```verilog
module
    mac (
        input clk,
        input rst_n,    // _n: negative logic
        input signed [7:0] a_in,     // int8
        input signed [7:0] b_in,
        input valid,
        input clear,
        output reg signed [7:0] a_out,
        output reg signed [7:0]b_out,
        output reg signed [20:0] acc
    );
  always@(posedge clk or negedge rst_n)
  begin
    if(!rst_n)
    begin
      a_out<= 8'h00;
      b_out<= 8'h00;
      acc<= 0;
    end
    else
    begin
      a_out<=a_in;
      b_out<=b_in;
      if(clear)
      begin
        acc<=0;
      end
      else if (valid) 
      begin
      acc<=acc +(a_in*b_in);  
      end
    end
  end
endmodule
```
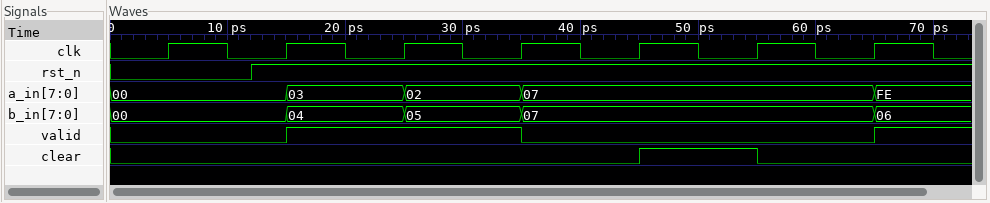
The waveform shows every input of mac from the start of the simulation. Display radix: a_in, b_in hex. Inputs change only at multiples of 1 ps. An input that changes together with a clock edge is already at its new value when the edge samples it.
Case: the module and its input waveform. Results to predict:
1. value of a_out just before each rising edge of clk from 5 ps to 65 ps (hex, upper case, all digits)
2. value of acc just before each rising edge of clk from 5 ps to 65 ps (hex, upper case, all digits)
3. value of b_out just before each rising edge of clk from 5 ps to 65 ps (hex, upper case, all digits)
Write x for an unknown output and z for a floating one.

00, 00, 03, 02, 07, 07, 07
000000, 000000, 00000C, 000016, 000016, 000000, 000000
00, 00, 04, 05, 07, 07, 07
